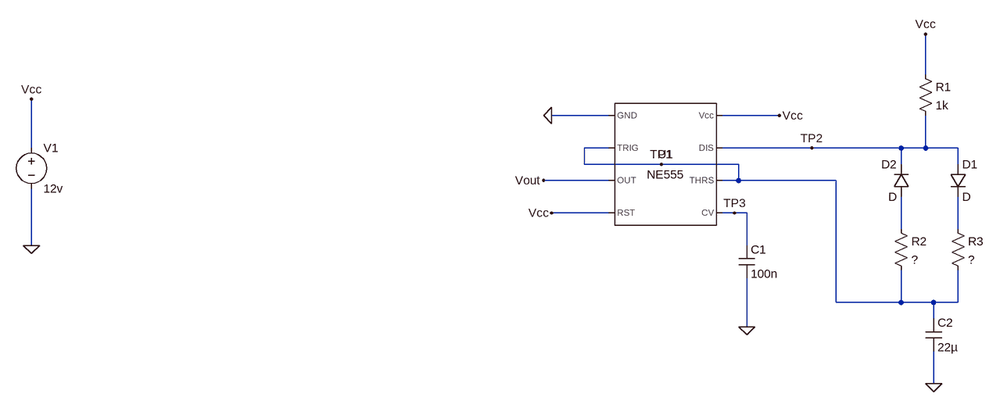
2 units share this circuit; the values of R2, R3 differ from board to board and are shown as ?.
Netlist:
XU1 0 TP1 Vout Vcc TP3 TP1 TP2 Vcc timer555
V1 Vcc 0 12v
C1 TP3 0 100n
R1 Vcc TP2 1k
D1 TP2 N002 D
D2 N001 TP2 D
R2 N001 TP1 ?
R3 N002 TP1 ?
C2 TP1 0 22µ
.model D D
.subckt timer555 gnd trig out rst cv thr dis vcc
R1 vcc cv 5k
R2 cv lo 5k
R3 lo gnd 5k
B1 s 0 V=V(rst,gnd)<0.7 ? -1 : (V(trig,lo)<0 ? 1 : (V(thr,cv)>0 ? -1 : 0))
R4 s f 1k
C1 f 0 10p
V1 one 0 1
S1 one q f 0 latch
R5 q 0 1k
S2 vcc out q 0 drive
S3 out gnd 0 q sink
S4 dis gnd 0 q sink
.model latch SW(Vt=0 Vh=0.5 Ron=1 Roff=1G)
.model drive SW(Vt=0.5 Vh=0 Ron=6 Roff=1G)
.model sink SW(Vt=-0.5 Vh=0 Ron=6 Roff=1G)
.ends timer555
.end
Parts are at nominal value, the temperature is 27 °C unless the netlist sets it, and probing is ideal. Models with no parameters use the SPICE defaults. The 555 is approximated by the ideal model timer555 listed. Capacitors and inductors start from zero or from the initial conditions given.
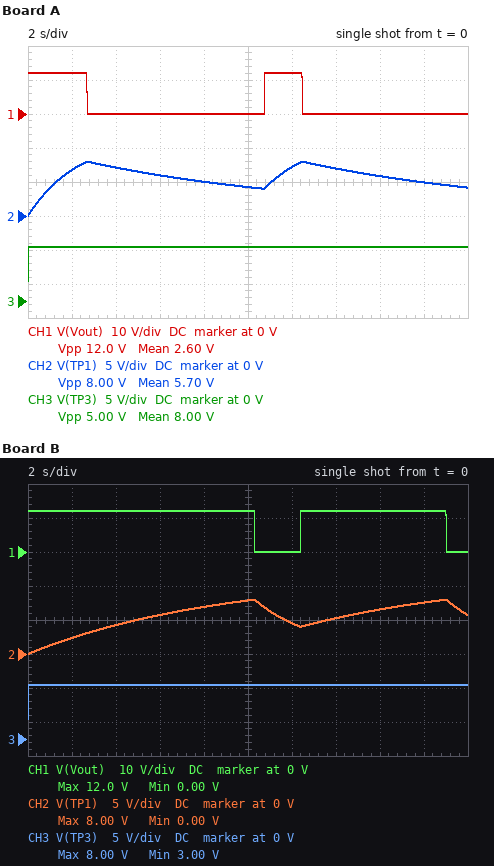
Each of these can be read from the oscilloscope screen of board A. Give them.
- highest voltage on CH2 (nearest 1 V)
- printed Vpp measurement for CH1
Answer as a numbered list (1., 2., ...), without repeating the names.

1. 8 V
2. 12.0 V
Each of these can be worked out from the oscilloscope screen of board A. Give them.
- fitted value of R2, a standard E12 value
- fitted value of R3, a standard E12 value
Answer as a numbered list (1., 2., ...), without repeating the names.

1. 470 kΩ
2. 100 kΩ
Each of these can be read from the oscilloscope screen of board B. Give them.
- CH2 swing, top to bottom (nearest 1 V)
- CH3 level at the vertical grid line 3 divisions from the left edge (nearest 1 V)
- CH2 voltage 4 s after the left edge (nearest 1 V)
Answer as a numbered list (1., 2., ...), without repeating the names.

1. 8 V
2. 8 V
3. 4 V
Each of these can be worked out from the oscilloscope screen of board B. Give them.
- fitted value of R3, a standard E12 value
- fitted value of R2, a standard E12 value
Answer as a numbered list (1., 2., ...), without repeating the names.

1. 390 kΩ
2. 120 kΩ
